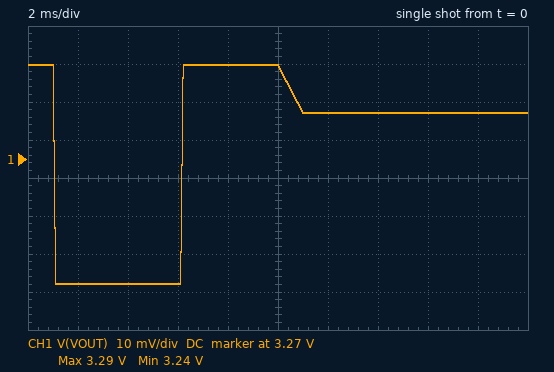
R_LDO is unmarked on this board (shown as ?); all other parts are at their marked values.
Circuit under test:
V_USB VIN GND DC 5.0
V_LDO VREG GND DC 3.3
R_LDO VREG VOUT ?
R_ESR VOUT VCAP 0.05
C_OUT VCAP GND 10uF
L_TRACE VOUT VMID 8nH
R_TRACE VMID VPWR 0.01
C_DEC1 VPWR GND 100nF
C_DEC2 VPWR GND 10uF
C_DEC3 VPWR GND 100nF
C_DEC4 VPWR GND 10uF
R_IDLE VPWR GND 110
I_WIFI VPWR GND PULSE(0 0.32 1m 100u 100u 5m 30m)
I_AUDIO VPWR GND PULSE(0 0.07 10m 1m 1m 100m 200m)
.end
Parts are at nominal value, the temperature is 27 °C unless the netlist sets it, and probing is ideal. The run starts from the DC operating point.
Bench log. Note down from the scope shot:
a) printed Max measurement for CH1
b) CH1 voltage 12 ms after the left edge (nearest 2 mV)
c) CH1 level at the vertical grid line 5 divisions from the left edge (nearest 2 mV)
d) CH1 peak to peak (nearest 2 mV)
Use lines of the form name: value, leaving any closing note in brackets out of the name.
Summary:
printed Max measurement for CH1: 3.29 V
CH1 voltage 12 ms after the left edge: 3.282 V
CH1 level at the vertical grid line 5 divisions from the left edge: 3.294 V
CH1 peak to peak: 58 mV
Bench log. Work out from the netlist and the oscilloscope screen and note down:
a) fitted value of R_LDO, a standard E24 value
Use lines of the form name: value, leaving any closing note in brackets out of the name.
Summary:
fitted value of R_LDO, a standard E24 value: 0.18 Ω
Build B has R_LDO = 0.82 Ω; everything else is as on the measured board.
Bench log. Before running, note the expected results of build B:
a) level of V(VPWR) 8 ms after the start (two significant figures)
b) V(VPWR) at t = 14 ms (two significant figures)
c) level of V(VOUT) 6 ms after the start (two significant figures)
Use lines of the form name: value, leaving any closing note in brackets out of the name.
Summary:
level of V(VPWR) 8 ms after the start: 3.3 V
V(VPWR) at t = 14 ms: 3.2 V
level of V(VOUT) 6 ms after the start: 3.0 V
